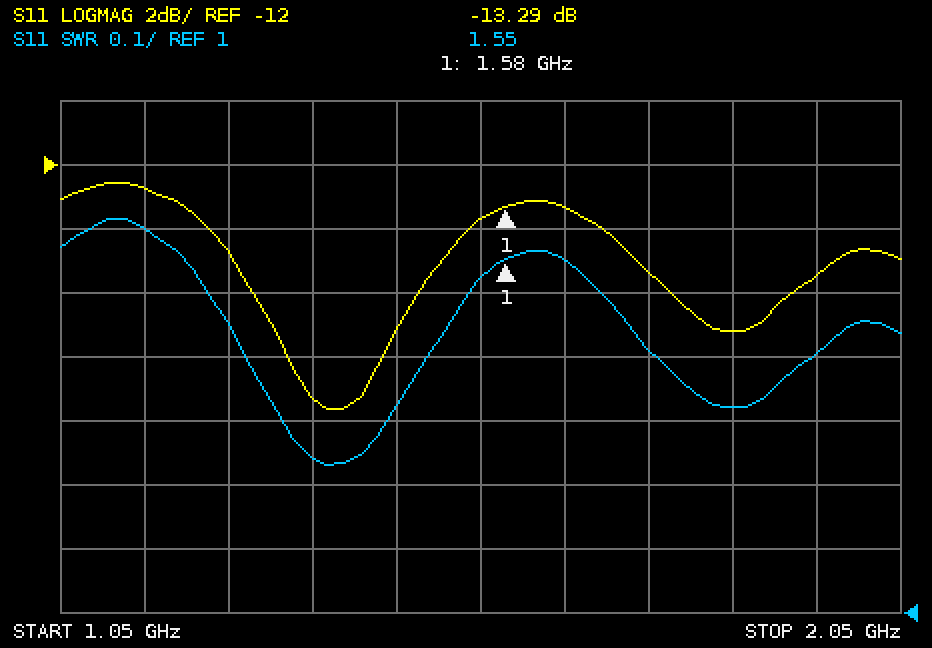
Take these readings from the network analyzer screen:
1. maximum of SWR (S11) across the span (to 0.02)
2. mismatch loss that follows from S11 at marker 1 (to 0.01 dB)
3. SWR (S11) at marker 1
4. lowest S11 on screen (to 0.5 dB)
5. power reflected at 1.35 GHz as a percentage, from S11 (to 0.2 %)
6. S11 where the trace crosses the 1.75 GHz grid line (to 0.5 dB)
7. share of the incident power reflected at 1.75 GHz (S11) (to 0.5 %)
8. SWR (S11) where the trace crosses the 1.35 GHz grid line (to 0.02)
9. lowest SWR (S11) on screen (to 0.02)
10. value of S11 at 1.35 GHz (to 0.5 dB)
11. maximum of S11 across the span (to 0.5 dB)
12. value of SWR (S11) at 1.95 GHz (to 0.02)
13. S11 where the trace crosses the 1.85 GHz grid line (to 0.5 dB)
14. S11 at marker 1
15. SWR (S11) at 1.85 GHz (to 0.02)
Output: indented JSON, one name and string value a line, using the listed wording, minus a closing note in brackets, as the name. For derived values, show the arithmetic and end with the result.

{
  "maximum of SWR (S11) across the span": "1.62",
  "mismatch loss that follows from S11 at marker 1": "−10 log10(1 − 10^(-13.29/10)) ≈ 0.21 dB",
  "SWR (S11) at marker 1": "1.55",
  "lowest S11 on screen": "-19.5 dB",
  "power reflected at 1.35 GHz as a percentage, from S11": "10^(-19.5/10) ≈ 1.12 %, so 1.2 % to the nearest 0.2 %",
  "S11 where the trace crosses the 1.75 GHz grid line": "-15.5 dB",
  "share of the incident power reflected at 1.75 GHz (S11)": "10^(-15.5/10) ≈ 2.82 %, so 3.0 % to the nearest 0.5 %",
  "SWR (S11) where the trace crosses the 1.35 GHz grid line": "1.24",
  "lowest SWR (S11) on screen": "1.24",
  "value of S11 at 1.35 GHz": "-19.5 dB",
  "maximum of S11 across the span": "-12.5 dB",
  "value of SWR (S11) at 1.95 GHz": "1.40",
  "S11 where the trace crosses the 1.85 GHz grid line": "-17.0 dB",
  "S11 at marker 1": "-13.29 dB",
  "SWR (S11) at 1.85 GHz": "1.32"
}
